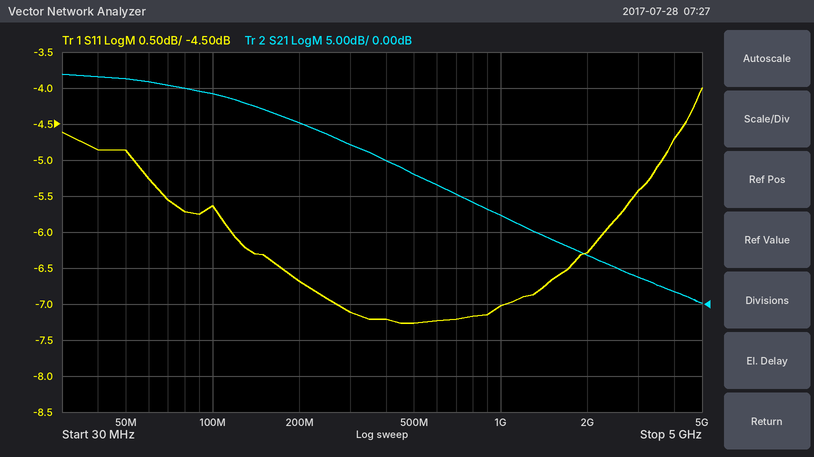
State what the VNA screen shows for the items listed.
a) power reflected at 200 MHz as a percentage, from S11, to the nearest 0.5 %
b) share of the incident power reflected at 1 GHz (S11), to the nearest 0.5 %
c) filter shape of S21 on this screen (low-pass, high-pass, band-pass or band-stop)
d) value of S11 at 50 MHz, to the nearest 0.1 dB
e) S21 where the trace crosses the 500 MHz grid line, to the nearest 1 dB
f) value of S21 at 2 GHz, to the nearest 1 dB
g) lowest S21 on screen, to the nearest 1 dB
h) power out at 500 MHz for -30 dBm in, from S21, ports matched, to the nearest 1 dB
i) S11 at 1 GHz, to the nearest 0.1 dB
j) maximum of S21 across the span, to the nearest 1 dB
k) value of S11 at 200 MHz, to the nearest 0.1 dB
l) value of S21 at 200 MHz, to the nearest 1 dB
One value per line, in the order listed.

21.5 %
20.0 %
low-pass
-4.9 dB
18 dB
7 dB
0 dB
-12 dBm
-7.0 dB
32 dB
-6.7 dB
25 dB
